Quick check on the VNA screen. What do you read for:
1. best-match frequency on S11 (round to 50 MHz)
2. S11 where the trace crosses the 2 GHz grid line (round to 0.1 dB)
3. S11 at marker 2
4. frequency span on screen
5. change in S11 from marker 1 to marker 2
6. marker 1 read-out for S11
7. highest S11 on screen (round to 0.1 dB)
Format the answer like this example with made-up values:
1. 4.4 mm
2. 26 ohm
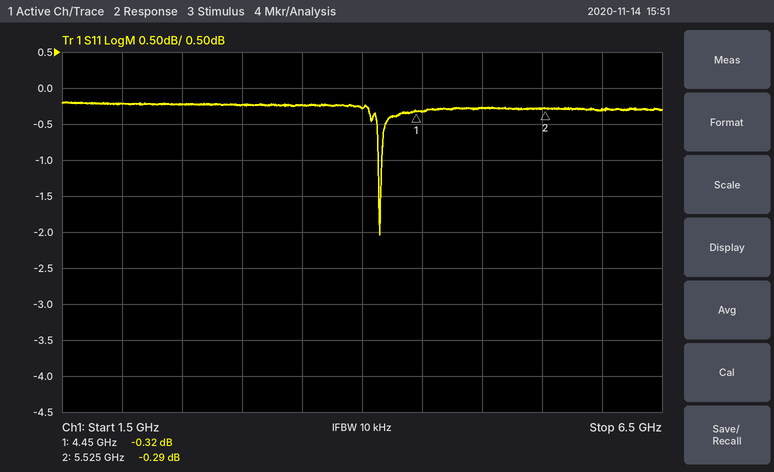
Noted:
1. 4.15 GHz
2. -0.2 dB
3. -0.29 dB
4. 5 GHz
5. 0.03 dB
6. -0.32 dB
7. -0.2 dB
